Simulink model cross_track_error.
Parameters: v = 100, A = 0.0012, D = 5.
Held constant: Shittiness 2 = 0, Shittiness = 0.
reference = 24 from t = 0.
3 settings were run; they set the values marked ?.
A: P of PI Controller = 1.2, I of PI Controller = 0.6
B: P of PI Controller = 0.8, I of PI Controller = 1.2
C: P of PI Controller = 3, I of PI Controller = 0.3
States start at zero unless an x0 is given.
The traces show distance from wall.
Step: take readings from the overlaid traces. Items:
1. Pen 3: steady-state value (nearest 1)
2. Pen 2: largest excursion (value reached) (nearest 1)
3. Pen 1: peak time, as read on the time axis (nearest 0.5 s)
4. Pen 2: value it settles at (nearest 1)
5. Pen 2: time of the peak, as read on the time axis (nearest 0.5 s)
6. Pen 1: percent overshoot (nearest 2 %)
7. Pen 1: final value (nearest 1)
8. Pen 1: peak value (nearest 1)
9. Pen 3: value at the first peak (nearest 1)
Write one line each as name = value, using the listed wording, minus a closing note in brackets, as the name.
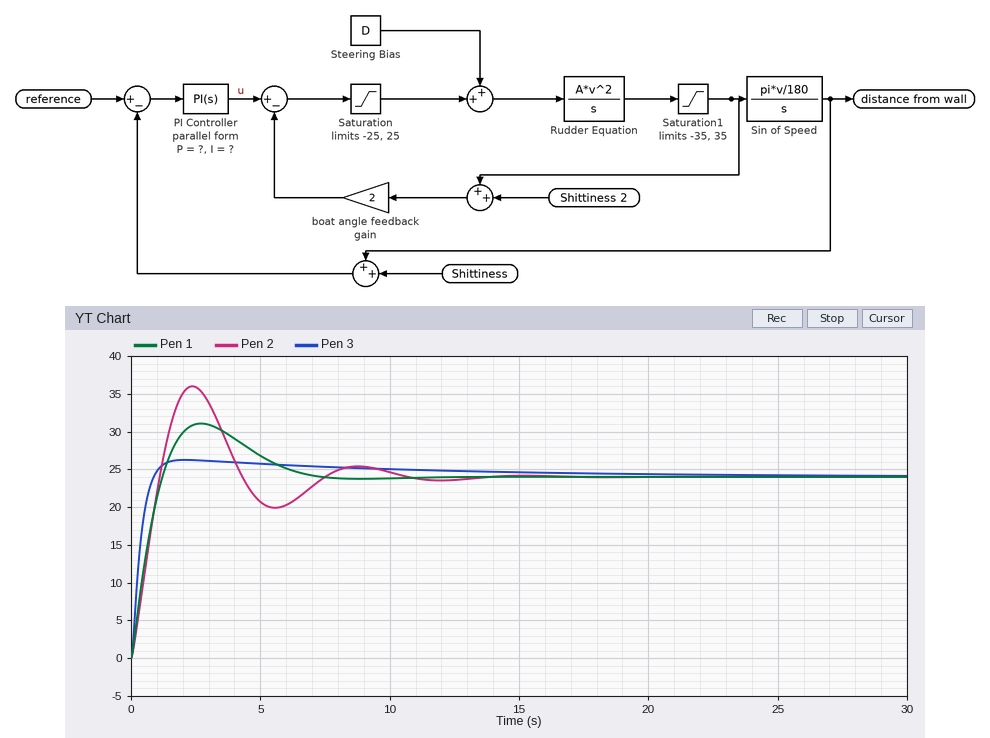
Pen 3: steady-state value = 24
Pen 2: largest excursion (value reached) = 36
Pen 1: peak time, as read on the time axis = 2.5 s
Pen 2: value it settles at = 24
Pen 2: time of the peak, as read on the time axis = 2.5 s
Pen 1: percent overshoot = 30 %
Pen 1: final value = 24
Pen 1: peak value = 31
Pen 3: value at the first peak = 26
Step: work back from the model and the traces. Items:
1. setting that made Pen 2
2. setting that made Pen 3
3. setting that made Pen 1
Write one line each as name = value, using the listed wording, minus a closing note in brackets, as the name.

setting that made Pen 2 = B
setting that made Pen 3 = C
setting that made Pen 1 = A
